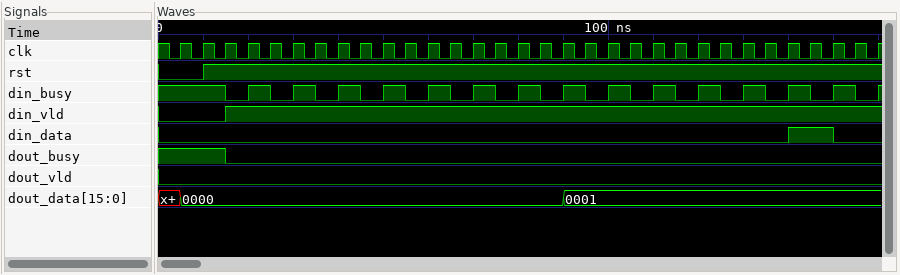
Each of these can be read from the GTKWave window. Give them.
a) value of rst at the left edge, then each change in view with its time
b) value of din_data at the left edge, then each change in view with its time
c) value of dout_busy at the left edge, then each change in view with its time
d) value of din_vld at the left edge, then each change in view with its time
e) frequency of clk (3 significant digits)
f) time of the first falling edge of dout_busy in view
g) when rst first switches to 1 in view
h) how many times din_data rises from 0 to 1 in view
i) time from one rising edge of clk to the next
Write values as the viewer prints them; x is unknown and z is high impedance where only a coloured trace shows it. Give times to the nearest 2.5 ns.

0, 1 at 10 ns
0, 1 at 140 ns, 0 at 150 ns
1, 0 at 15 ns
0, 1 at 15 ns
200 MHz
15 ns
10 ns
1
5 ns
